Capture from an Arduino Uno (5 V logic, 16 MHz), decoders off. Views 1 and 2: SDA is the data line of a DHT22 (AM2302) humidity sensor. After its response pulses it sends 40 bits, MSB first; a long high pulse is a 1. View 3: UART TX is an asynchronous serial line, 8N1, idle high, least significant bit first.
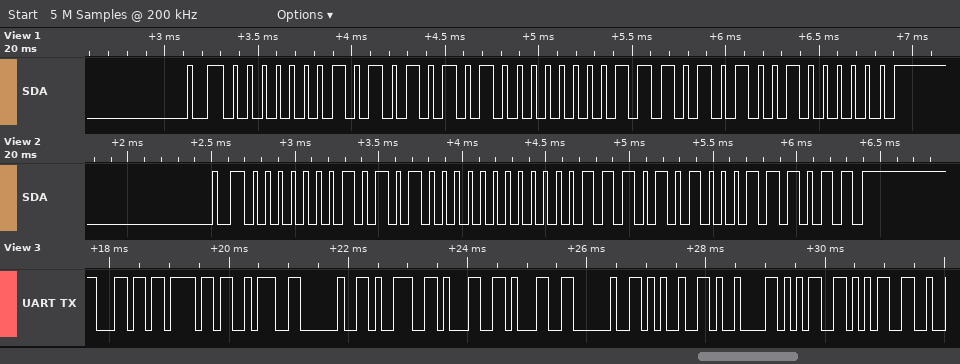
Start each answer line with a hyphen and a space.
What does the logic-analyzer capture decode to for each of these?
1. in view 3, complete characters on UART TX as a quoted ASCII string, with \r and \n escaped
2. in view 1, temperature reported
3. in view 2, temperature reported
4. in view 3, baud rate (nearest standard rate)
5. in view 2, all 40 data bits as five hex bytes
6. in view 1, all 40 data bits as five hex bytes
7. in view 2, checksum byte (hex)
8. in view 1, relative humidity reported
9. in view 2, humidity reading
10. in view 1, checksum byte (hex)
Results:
- "lo: 911 %\t55"
- 23.4 °C
- 23.4 °C
- 9600 baud
- 01 50 00 EA 3B
- 01 55 00 EA 40
- 0x3B
- 34.1 %
- 33.6 %
- 0x40
